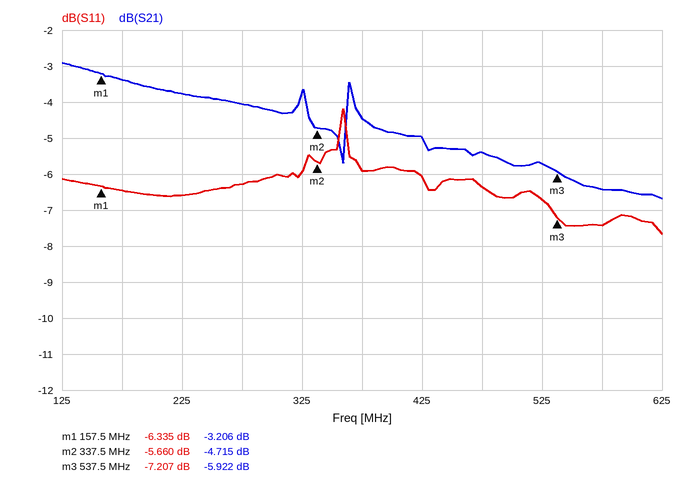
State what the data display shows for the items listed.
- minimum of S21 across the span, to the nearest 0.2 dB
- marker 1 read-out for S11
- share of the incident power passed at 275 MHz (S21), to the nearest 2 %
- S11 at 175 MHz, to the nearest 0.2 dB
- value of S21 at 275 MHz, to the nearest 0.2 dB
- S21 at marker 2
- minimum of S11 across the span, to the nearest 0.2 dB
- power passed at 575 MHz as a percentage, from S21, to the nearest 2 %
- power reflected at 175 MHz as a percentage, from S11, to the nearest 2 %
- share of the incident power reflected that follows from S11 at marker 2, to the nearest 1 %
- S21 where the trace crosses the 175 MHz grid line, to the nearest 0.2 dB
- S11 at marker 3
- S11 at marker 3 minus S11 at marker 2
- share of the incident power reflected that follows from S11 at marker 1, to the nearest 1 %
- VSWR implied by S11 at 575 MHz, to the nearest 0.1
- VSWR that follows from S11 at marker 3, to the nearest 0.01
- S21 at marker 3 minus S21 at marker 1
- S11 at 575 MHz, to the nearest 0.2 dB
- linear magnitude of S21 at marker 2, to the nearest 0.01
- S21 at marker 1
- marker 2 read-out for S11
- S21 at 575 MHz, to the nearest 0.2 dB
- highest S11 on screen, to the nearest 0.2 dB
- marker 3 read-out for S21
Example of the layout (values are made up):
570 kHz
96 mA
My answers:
-6.6 dB
-6.335 dB
40 %
-6.4 dB
-4.0 dB
-4.715 dB
-7.6 dB
22 %
22 %
27 %
-3.4 dB
-7.207 dB
-1.547 dB
23 %
2.5
2.55
-2.716 dB
-7.4 dB
0.58
-3.206 dB
-5.660 dB
-6.4 dB
-4.2 dB
-5.922 dB
